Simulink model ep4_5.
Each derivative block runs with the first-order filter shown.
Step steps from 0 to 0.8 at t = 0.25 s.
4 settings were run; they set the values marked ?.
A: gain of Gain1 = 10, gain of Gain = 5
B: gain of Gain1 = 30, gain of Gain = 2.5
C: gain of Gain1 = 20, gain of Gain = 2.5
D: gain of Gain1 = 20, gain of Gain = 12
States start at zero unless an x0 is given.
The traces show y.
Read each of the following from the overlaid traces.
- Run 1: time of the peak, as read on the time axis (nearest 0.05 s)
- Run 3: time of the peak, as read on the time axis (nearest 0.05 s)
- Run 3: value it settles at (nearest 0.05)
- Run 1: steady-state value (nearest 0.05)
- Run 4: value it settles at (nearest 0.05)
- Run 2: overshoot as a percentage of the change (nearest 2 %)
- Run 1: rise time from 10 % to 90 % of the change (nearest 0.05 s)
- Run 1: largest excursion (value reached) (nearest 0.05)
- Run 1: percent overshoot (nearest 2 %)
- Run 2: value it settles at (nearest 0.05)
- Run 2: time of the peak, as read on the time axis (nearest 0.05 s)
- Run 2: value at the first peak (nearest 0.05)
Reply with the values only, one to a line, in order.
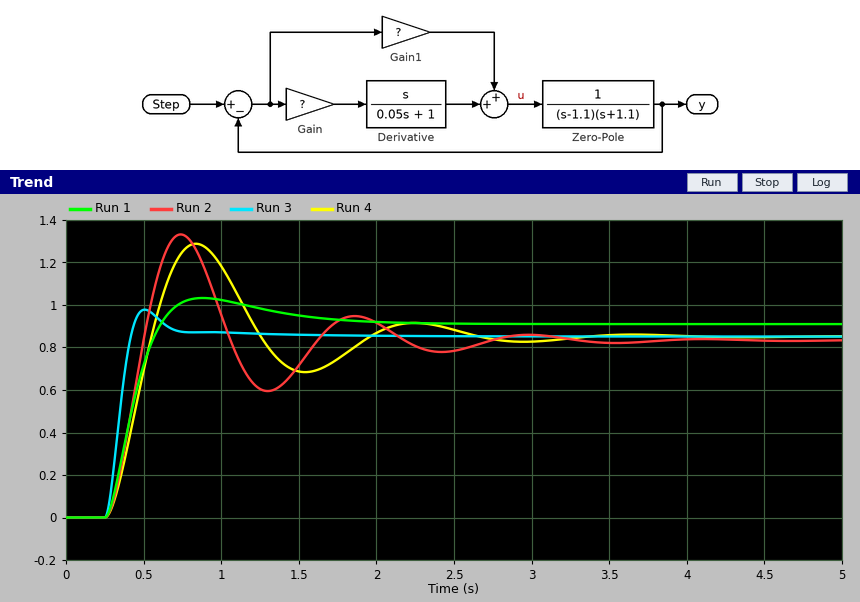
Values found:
0.90 s
0.50 s
0.85
0.90
0.85
60 %
0.25 s
1.05
14 %
0.85
0.75 s
1.35
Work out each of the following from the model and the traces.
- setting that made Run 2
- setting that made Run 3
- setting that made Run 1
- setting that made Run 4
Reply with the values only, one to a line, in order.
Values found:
B
D
A
C
